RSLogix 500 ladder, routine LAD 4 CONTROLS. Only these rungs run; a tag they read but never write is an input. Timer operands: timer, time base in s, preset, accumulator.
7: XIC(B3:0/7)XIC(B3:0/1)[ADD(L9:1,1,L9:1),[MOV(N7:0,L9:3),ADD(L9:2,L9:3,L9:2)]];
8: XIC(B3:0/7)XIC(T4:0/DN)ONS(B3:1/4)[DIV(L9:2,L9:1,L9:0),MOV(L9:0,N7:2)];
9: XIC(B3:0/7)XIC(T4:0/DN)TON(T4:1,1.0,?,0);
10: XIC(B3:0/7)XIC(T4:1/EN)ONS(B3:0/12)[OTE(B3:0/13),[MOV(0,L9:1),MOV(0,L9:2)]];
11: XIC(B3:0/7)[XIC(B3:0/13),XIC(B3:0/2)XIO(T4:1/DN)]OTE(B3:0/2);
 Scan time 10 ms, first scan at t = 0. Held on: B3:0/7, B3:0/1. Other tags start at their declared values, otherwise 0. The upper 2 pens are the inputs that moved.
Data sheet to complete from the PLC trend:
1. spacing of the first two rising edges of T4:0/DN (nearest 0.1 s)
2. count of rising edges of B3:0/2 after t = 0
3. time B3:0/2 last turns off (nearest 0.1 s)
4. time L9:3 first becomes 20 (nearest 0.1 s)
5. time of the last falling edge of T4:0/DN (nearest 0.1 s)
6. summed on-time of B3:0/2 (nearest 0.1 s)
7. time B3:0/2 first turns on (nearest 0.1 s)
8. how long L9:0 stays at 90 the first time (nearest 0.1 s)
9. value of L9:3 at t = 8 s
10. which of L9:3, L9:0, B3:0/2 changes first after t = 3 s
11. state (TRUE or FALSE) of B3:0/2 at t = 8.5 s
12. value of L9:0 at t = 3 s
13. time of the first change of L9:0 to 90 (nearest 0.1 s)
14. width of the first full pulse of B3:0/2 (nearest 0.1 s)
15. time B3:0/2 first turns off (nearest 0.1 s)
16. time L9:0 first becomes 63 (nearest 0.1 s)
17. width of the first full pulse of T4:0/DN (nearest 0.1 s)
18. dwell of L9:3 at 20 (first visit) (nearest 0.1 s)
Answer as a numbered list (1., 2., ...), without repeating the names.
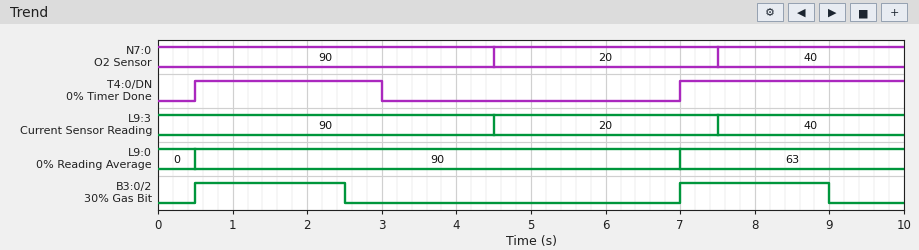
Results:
1. 6.5 s
2. 2
3. 9.0 s
4. 4.5 s
5. 3.0 s
6. 4.0 s
7. 0.5 s
8. 6.5 s
9. 40
10. L9:3
11. TRUE
12. 90
13. 0.5 s
14. 2.0 s
15. 2.5 s
16. 7.0 s
17. 2.5 s
18. 3.0 s
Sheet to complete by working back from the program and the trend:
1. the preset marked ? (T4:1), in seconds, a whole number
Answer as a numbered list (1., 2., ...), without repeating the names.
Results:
1. 2 s
